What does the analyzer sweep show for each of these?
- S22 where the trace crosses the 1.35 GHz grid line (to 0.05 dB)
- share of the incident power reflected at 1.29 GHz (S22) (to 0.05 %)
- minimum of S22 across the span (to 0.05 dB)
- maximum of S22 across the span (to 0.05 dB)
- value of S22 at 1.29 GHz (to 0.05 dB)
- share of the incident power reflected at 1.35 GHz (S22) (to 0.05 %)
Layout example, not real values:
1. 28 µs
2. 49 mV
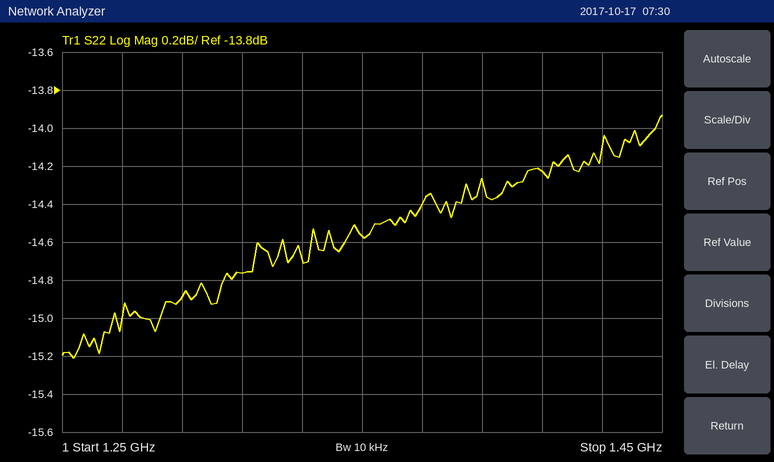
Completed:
1. -14.55 dB
2. 3.25 %
3. -15.20 dB
4. -13.95 dB
5. -14.90 dB
6. 3.50 %
